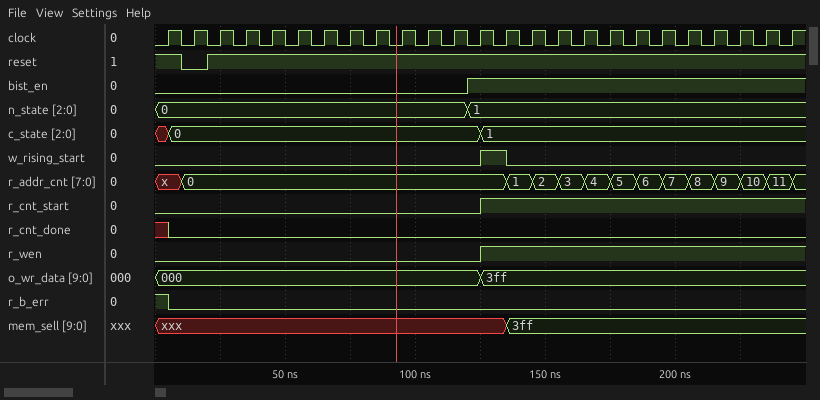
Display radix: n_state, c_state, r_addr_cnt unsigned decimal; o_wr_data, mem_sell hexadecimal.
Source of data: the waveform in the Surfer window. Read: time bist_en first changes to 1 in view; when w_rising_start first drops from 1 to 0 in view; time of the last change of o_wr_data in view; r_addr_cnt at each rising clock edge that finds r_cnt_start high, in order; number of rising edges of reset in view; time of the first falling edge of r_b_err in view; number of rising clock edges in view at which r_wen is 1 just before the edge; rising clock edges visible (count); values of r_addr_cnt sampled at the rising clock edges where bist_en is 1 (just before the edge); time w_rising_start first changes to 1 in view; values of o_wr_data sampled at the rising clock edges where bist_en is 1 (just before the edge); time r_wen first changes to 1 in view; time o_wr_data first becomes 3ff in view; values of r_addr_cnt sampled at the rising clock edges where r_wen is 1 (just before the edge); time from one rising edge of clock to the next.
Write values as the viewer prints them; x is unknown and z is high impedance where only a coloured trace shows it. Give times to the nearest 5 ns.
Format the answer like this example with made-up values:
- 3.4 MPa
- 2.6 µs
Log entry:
- 120 ns
- 135 ns
- 125 ns
- 0, 1, 2, 3, 4, 5, 6, 7, 8, 9, 10, 11
- 1
- 5 ns
- 12
- 25
- 0, 0, 1, 2, 3, 4, 5, 6, 7, 8, 9, 10, 11
- 125 ns
- 000, 3ff, 3ff, 3ff, 3ff, 3ff, 3ff, 3ff, 3ff, 3ff, 3ff, 3ff, 3ff
- 125 ns
- 125 ns
- 0, 1, 2, 3, 4, 5, 6, 7, 8, 9, 10, 11
- 10 ns
